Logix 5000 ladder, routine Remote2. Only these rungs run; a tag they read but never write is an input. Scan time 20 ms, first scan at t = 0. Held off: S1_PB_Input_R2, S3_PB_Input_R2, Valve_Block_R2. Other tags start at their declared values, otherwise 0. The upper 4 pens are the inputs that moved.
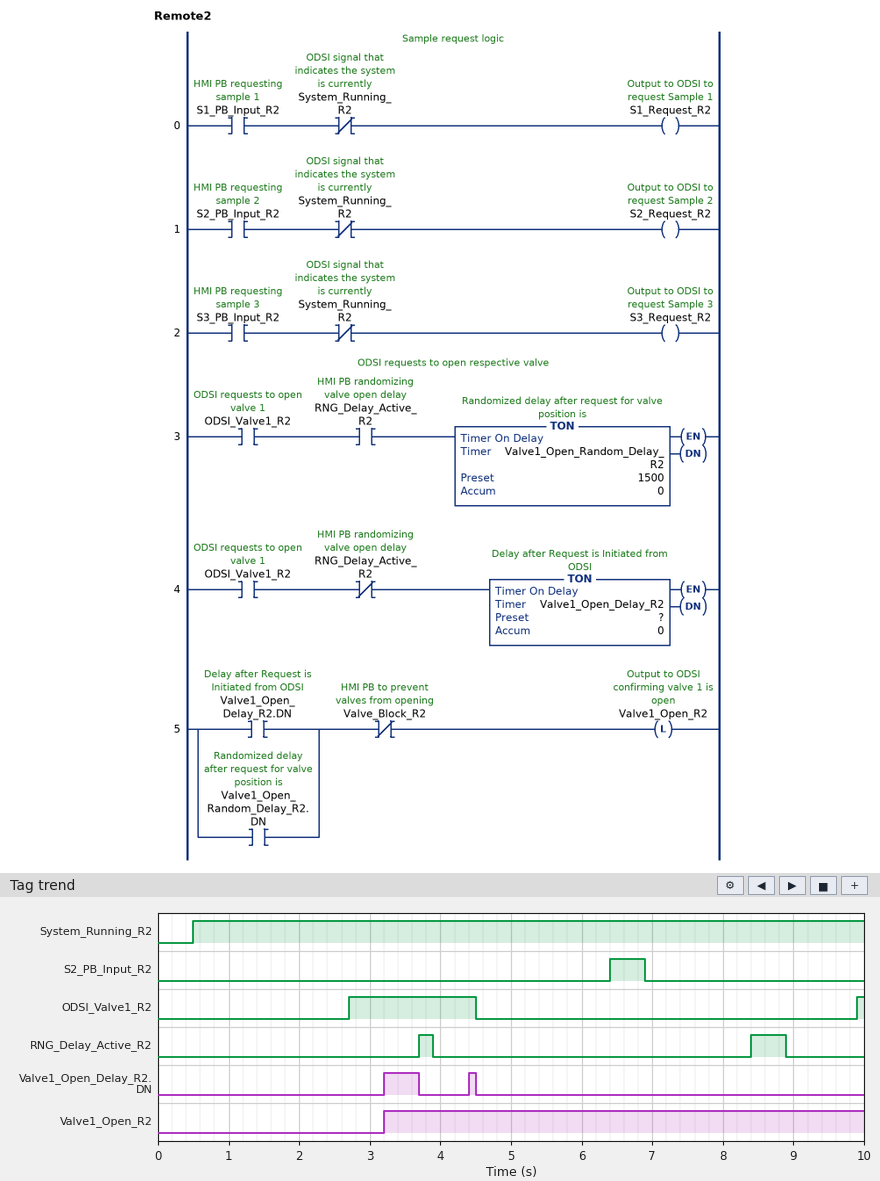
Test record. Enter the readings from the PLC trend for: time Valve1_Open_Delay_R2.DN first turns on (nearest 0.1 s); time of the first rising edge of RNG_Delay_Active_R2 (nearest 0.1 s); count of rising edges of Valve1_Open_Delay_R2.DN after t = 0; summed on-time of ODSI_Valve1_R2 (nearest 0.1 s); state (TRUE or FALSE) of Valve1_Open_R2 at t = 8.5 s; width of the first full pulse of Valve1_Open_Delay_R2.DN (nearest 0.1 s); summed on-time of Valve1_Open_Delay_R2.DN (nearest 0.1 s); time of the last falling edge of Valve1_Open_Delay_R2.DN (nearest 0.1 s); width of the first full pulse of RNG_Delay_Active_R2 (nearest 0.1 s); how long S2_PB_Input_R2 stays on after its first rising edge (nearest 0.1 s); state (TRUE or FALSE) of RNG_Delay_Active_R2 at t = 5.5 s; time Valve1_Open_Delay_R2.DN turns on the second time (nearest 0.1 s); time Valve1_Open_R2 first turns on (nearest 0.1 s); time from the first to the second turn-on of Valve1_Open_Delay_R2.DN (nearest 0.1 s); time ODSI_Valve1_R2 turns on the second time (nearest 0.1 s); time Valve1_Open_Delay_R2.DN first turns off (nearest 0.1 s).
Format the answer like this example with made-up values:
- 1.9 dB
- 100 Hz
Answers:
- 3.2 s
- 3.7 s
- 2
- 1.9 s
- TRUE
- 0.5 s
- 0.6 s
- 4.5 s
- 0.2 s
- 0.5 s
- FALSE
- 4.4 s
- 3.2 s
- 1.2 s
- 9.9 s
- 3.7 s
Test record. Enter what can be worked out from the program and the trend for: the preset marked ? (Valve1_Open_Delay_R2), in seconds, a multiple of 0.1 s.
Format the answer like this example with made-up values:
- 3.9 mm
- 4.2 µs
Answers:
- 0.5 s
